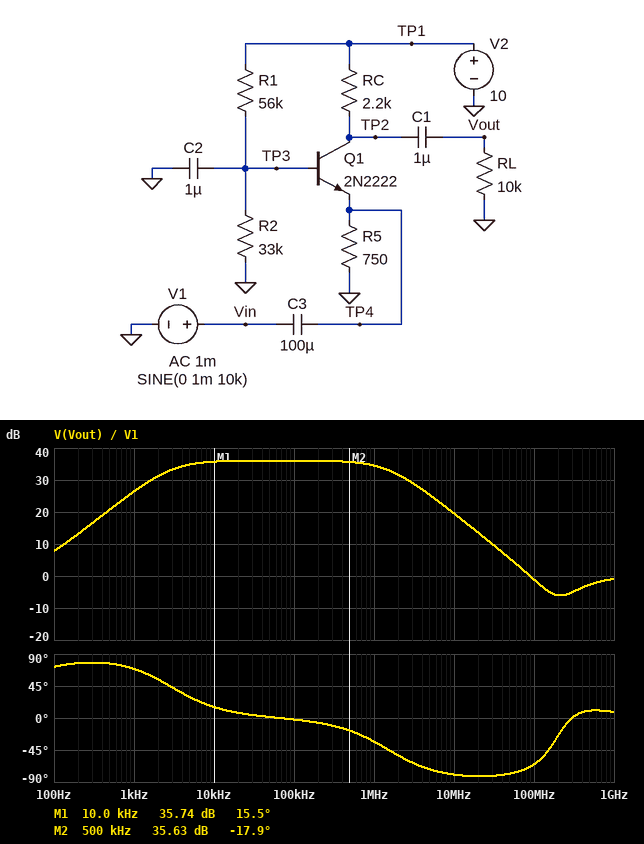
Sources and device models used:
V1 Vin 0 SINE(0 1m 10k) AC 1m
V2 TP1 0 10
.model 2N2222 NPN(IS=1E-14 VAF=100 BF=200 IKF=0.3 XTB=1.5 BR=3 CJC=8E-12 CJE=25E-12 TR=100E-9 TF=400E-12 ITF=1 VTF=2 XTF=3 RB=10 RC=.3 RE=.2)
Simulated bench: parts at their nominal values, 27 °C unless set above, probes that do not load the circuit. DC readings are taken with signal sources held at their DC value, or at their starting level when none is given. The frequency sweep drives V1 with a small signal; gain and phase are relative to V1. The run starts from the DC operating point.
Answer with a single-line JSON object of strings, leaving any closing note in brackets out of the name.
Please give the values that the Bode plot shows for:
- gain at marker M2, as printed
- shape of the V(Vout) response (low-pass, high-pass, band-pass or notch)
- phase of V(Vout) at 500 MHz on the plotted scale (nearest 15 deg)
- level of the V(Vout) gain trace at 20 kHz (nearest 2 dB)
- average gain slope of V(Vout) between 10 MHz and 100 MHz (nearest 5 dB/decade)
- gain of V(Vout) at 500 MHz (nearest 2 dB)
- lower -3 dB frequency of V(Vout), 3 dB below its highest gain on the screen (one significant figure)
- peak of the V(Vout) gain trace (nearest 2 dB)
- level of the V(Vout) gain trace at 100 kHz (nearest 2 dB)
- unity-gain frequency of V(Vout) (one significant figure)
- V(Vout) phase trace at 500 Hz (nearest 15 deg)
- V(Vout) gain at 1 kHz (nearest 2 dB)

{"gain at marker M2, as printed": "35.63 dB", "shape of the V(Vout) response": "band-pass", "phase of V(Vout) at 500 MHz on the plotted scale": "15 deg", "level of the V(Vout) gain trace at 20 kHz": "36 dB", "average gain slope of V(Vout) between 10 MHz and 100 MHz": "-20 dB/decade", "gain of V(Vout) at 500 MHz": "-2 dB", "lower -3 dB frequency of V(Vout), 3 dB below its highest gain on the screen": "3 kHz", "peak of the V(Vout) gain trace": "36 dB", "level of the V(Vout) gain trace at 100 kHz": "36 dB", "unity-gain frequency of V(Vout)": "90 MHz", "V(Vout) phase trace at 500 Hz": "75 deg", "V(Vout) gain at 1 kHz": "26 dB"}
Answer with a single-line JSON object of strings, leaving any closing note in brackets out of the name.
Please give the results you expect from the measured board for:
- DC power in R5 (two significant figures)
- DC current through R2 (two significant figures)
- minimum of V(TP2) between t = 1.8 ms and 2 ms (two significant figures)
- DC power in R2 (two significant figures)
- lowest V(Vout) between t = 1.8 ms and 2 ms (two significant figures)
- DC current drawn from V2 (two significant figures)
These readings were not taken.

{"DC power in R5": "8.5 mW", "DC current through R2": "97 µA", "minimum of V(TP2) between t = 1.8 ms and 2 ms": "2.6 V", "DC power in R2": "310 µW", "lowest V(Vout) between t = 1.8 ms and 2 ms": "-40 mV", "DC current drawn from V2": "3.5 mA"}
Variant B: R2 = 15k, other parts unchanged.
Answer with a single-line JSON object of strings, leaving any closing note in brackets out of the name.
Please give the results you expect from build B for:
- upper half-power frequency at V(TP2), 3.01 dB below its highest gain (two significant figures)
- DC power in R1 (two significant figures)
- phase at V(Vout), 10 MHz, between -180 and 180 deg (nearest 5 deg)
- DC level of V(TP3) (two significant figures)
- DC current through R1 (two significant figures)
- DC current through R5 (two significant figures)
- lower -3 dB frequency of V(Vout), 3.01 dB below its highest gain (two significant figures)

{"upper half-power frequency at V(TP2), 3.01 dB below its highest gain": "12 MHz", "DC power in R1": "1.1 mW", "phase at V(Vout), 10 MHz, between -180 and 180 deg": "-40 deg", "DC level of V(TP3)": "2.0 V", "DC current through R1": "140 µA", "DC current through R5": "1.8 mA", "lower -3 dB frequency of V(Vout), 3.01 dB below its highest gain": "160 Hz"}
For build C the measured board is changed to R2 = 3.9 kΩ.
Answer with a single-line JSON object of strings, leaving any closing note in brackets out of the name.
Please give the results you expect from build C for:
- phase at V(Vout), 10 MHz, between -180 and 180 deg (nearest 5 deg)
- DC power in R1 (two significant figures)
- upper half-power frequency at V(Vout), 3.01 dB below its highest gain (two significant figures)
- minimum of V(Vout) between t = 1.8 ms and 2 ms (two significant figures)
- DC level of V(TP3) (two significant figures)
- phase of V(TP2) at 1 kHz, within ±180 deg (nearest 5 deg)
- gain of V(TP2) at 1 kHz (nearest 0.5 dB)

{"phase at V(Vout), 10 MHz, between -180 and 180 deg": "-25 deg", "DC power in R1": "1.6 mW", "upper half-power frequency at V(Vout), 3.01 dB below its highest gain": "24 MHz", "minimum of V(Vout) between t = 1.8 ms and 2 ms": "-5.8 mV", "DC level of V(TP3)": "650 mV", "phase of V(TP2) at 1 kHz, within ±180 deg": "0 deg", "gain of V(TP2) at 1 kHz": "15.0 dB"}
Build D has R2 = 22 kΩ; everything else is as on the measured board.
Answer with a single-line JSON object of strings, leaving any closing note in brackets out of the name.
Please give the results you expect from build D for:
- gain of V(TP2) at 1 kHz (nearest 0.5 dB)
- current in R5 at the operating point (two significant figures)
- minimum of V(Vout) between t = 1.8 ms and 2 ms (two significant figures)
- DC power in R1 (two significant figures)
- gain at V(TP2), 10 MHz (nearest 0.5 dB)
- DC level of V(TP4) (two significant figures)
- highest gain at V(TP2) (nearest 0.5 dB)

{"gain of V(TP2) at 1 kHz": "44.0 dB", "current in R5 at the operating point": "2.6 mA", "minimum of V(Vout) between t = 1.8 ms and 2 ms": "-170 mV", "DC power in R1": "970 µW", "gain at V(TP2), 10 MHz": "40.5 dB", "DC level of V(TP4)": "1.9 V", "highest gain at V(TP2)": "44.5 dB"}
